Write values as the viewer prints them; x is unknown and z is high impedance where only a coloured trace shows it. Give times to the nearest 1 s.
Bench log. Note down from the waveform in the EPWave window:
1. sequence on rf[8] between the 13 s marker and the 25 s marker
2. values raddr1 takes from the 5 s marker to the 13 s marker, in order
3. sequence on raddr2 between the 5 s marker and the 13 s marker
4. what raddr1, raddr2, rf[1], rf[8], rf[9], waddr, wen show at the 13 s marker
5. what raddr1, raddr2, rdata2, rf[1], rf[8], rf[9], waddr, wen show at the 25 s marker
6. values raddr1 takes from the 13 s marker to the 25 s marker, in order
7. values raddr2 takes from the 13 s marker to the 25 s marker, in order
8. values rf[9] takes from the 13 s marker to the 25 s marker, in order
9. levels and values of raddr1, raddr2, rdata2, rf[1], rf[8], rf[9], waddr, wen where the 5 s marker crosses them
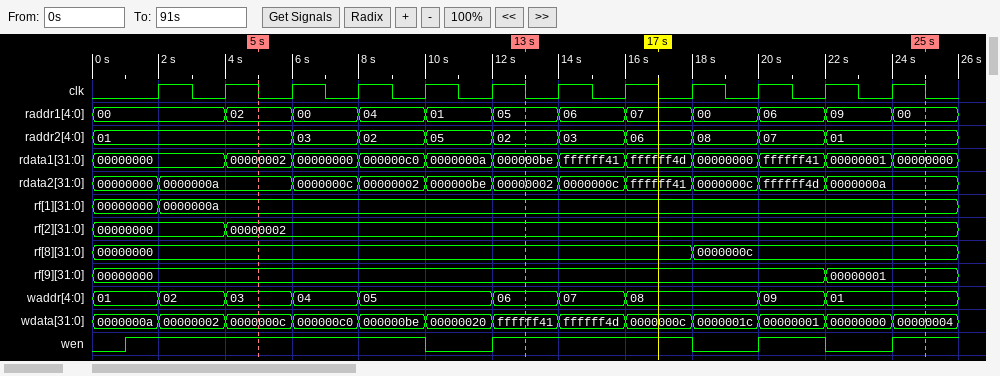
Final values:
00000000, 0000000c
02, 00, 04, 01, 05
01, 03, 02, 05, 02
raddr1=05, raddr2=02, rf[1]=0000000a, rf[8]=00000000, rf[9]=00000000, waddr=06, wen=1
raddr1=00, raddr2=01, rdata2=0000000a, rf[1]=0000000a, rf[8]=0000000c, rf[9]=00000001, waddr=01, wen=1
05, 06, 07, 00, 06, 09, 00
02, 03, 06, 08, 07, 01
00000000, 00000001
raddr1=02, raddr2=01, rdata2=0000000a, rf[1]=0000000a, rf[8]=00000000, rf[9]=00000000, waddr=03, wen=1
